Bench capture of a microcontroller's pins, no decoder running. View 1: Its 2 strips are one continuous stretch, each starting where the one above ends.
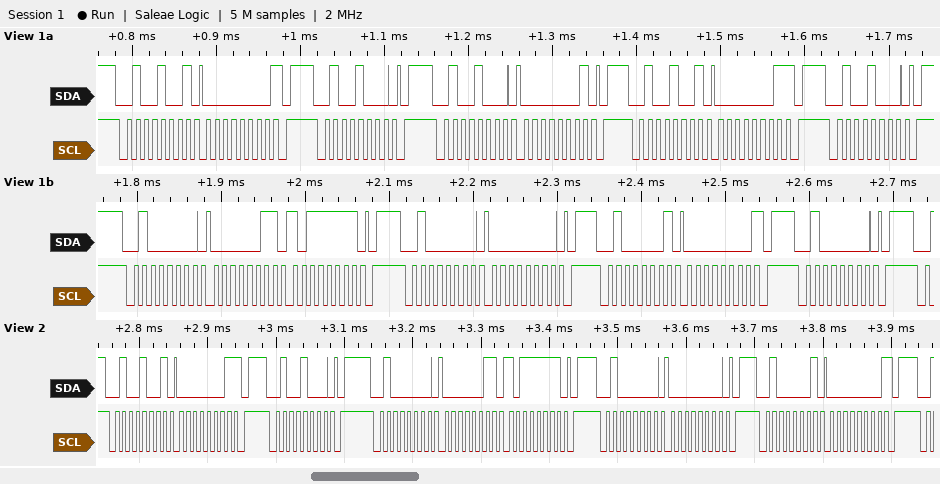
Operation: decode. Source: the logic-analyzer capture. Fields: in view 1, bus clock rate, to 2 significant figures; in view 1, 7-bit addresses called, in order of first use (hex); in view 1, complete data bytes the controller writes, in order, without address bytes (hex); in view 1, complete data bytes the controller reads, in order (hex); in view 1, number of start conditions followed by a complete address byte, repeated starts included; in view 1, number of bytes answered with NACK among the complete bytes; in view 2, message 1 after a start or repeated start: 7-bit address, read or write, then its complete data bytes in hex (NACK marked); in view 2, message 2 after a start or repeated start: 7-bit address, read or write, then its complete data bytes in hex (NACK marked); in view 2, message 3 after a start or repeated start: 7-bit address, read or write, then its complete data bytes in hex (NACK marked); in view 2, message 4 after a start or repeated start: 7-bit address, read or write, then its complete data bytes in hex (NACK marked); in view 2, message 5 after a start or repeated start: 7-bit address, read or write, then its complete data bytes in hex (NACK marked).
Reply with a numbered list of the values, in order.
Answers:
1. 100 kHz
2. 0x24 0x20
3. 01 03 BF 00
4. 00 01 00
5. 9
6. 3
7. 0x24 read: 01 NACK
8. 0x24 write
9. 0x20 write: 03 BF
10. 0x20 write: 00
11. 0x20 read: 00 NACK
